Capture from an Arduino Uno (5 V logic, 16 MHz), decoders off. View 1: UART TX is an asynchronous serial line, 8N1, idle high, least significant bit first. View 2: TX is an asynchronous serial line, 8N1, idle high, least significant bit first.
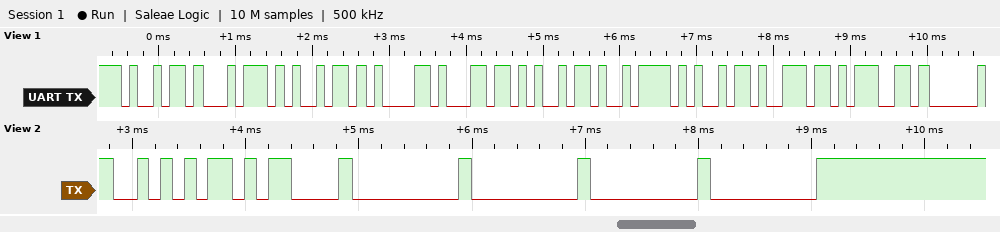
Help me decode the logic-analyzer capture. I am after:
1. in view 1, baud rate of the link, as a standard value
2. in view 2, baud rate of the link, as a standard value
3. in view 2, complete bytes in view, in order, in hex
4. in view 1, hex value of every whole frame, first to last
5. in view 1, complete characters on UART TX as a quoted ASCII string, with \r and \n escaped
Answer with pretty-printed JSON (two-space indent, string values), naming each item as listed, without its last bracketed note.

{
  "in view 1, baud rate of the link, as a standard value": "9600 baud",
  "in view 2, baud rate of the link, as a standard value": "9600 baud",
  "in view 2, complete bytes in view, in order, in hex": "AA 0D 00 00 00 00",
  "in view 1, hex value of every whole frame, first to last": "69 74 69 61 6C 69 7A 69 6E 67",
  "in view 1, complete characters on UART TX as a quoted ASCII string, with \\r and \\n escaped": "\"itializing\""
}
